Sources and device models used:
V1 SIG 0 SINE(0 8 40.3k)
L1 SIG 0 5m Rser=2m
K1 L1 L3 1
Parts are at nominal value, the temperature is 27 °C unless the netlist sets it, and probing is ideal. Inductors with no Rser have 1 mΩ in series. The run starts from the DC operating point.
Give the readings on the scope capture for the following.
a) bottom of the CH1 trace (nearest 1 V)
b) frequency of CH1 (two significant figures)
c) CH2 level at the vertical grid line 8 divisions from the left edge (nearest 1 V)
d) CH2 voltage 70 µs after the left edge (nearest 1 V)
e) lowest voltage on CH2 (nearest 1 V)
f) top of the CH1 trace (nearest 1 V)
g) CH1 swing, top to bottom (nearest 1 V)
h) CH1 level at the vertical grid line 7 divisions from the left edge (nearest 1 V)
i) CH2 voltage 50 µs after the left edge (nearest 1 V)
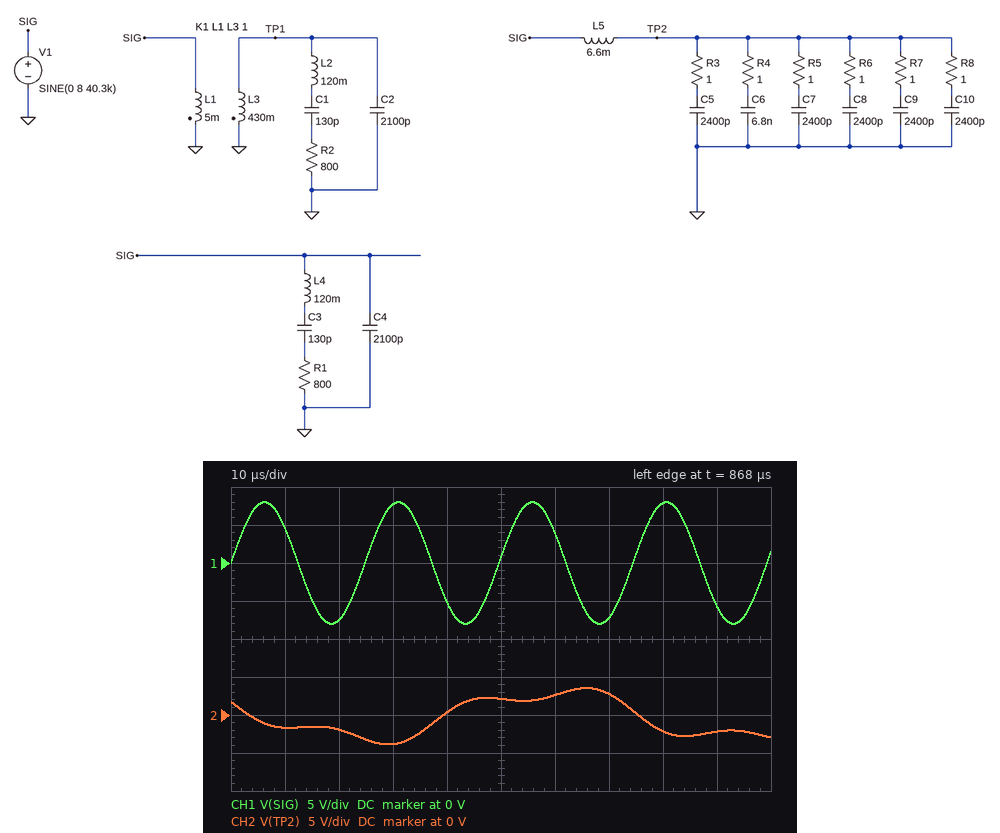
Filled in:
-8 V
40 kHz
-2 V
3 V
-4 V
8 V
16 V
-7 V
2 V
